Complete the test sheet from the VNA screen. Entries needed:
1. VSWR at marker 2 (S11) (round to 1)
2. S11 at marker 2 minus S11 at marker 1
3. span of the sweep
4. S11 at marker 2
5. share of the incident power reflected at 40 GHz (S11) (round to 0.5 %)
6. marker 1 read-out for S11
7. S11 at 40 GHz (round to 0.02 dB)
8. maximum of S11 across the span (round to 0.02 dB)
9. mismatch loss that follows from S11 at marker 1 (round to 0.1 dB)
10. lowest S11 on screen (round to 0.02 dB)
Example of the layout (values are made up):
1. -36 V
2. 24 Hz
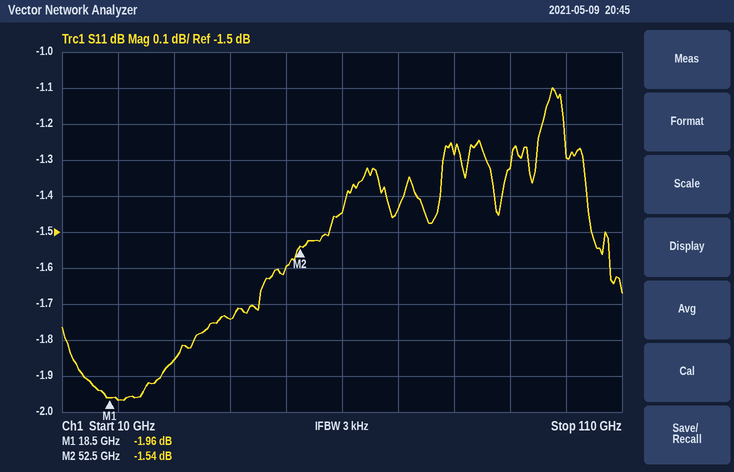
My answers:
1. 11
2. 0.42 dB
3. 100 GHz
4. -1.54 dB
5. 67.0 %
6. -1.96 dB
7. -1.74 dB
8. -1.10 dB
9. 4.4 dB
10. -1.96 dB
